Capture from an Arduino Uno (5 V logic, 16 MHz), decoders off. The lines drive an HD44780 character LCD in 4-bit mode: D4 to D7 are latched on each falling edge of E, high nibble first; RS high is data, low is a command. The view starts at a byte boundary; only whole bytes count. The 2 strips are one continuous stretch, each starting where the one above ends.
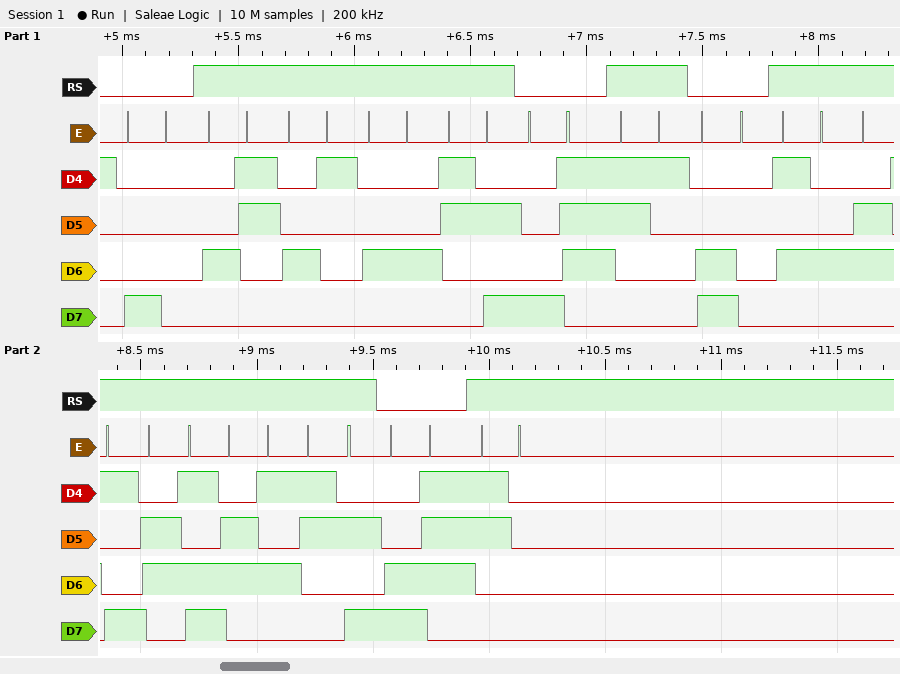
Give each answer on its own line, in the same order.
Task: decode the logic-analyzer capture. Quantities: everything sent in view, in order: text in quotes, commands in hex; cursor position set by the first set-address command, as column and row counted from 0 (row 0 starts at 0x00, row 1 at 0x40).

0x80 "CAD:" 0x87 "1" 0xC0 "Time:" 0xC7 "0"
column 0, row 0
